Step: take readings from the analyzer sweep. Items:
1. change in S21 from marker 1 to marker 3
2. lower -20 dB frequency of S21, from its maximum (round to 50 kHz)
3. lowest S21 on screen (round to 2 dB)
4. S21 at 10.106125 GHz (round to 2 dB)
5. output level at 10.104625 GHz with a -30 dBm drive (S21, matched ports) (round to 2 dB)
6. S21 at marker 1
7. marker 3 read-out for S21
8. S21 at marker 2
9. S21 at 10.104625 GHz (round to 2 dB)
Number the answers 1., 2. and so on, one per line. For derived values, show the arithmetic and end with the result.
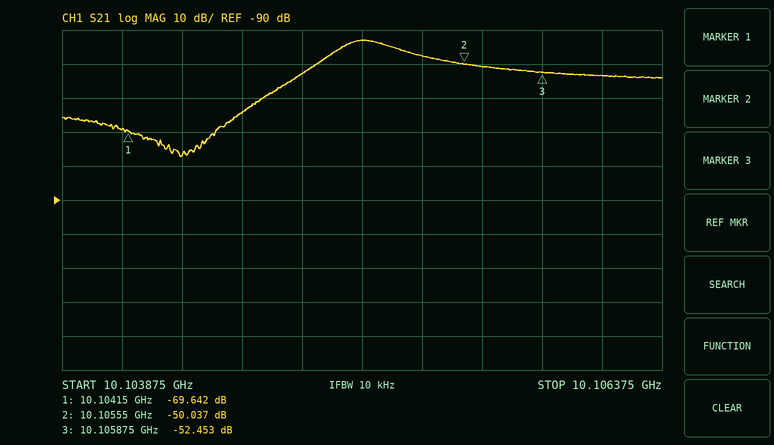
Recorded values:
1. -52.453 − (-69.642) = 17.189 dB
2. 10.10465 GHz
3. -78 dB
4. -54 dB
5. -30 dBm + (-64 dB) = -94 dBm
6. -69.642 dB
7. -52.453 dB
8. -50.037 dB
9. -64 dB
